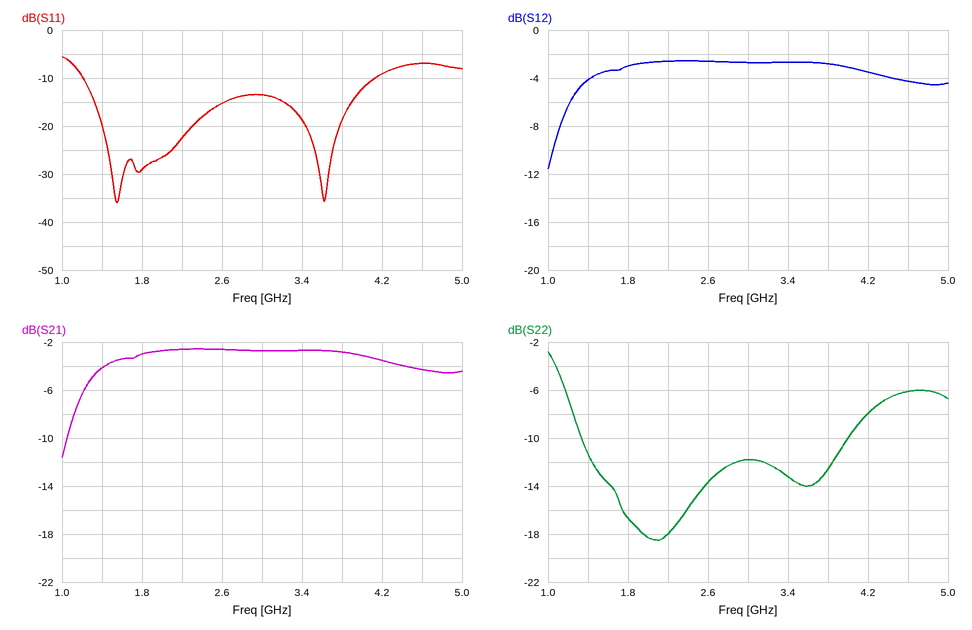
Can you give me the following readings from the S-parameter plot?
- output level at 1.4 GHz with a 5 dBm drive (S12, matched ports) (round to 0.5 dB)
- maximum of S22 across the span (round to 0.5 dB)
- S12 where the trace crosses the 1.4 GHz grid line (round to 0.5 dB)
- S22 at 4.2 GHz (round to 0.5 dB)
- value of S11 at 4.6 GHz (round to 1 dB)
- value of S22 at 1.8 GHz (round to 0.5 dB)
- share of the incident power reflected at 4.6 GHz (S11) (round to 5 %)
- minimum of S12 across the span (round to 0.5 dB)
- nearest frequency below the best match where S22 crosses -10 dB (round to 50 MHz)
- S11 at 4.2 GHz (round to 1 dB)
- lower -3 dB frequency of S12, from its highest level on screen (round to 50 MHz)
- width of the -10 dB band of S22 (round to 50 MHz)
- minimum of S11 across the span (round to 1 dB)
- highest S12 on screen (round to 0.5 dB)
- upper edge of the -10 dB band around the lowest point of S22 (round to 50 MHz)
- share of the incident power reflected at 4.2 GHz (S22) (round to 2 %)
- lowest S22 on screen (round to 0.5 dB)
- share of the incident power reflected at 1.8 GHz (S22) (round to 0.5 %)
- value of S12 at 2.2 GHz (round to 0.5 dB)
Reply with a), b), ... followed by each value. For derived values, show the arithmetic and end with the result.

a) 5 dBm + (-4.0 dB) = 1.0 dBm
b) -3.0 dB
c) -4.0 dB
d) -8.0 dB
e) -7 dB
f) -16.5 dB
g) 10^(-7/10) ≈ 20 %
h) -11.5 dB
i) 1.35 GHz
j) -9 dB
k) 1.25 GHz
l) 4.00 GHz − 1.35 GHz = 2.65 GHz
m) -36 dB
n) -2.5 dB
o) 4.00 GHz
p) 10^(-8/10) ≈ 16 %
q) -18.5 dB
r) 10^(-16.5/10) ≈ 2.24 %, so 2.0 % to the nearest 0.5 %
s) -2.5 dB
